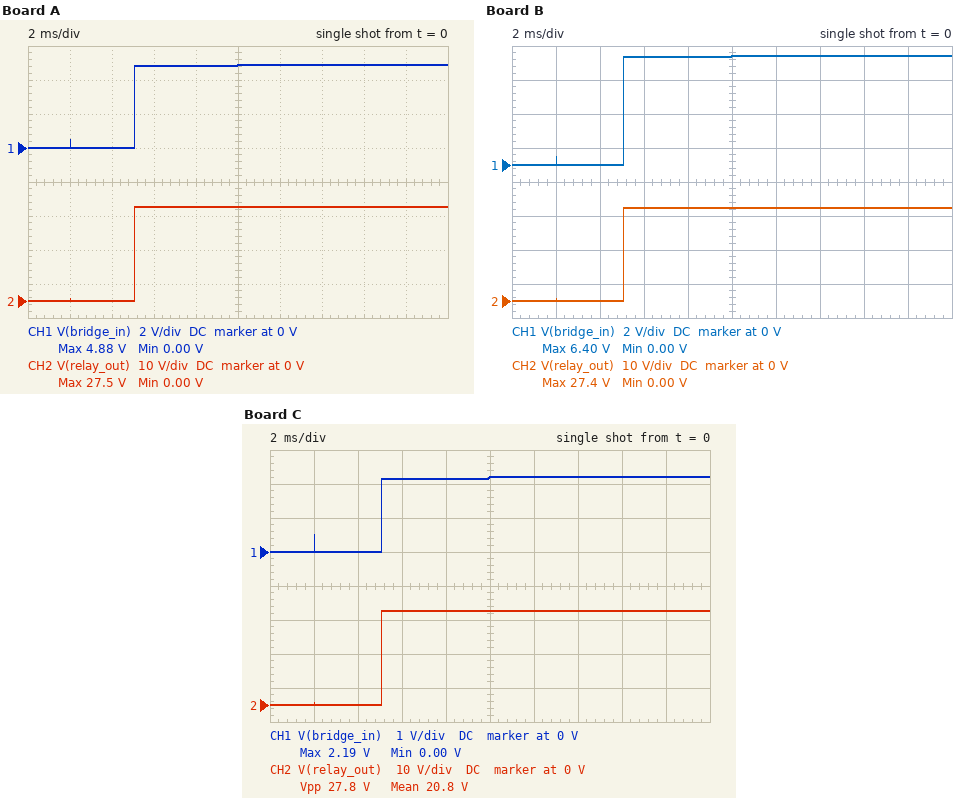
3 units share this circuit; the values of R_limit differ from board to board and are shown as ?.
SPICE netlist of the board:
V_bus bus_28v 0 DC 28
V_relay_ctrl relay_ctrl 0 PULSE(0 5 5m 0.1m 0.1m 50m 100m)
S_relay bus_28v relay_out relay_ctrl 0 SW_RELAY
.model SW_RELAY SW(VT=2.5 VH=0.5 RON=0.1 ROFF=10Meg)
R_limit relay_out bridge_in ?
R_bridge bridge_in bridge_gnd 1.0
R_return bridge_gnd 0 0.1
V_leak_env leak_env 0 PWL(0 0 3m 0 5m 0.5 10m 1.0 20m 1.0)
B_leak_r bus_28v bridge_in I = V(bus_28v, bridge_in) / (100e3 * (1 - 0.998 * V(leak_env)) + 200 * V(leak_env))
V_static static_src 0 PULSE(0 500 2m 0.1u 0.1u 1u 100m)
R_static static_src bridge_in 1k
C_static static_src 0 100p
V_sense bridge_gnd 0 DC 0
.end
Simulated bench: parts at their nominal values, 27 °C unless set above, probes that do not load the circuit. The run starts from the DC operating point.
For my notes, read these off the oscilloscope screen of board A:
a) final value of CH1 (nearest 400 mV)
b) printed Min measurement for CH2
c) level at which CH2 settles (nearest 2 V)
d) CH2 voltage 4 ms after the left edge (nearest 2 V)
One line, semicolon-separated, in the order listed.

4.8 V; 0.00 V; 28 V; 0 V
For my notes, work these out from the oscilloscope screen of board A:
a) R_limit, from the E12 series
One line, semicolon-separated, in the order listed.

4.7 Ω
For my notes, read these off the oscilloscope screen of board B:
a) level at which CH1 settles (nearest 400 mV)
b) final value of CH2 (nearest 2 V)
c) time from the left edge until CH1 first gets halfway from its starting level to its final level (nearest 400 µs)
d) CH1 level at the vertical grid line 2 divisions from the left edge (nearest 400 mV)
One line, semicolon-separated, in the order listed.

6.4 V; 28 V; 5.2 ms; 0 V
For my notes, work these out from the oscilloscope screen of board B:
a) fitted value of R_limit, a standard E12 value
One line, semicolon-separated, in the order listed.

3.3 Ω
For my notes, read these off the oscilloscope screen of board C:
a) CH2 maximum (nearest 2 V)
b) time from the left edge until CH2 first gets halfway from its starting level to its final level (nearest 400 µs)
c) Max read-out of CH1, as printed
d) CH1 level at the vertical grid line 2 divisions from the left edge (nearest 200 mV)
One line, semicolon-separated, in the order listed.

28 V; 5.2 ms; 2.19 V; 0 V
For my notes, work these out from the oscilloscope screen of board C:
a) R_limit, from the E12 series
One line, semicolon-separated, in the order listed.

12 Ω
